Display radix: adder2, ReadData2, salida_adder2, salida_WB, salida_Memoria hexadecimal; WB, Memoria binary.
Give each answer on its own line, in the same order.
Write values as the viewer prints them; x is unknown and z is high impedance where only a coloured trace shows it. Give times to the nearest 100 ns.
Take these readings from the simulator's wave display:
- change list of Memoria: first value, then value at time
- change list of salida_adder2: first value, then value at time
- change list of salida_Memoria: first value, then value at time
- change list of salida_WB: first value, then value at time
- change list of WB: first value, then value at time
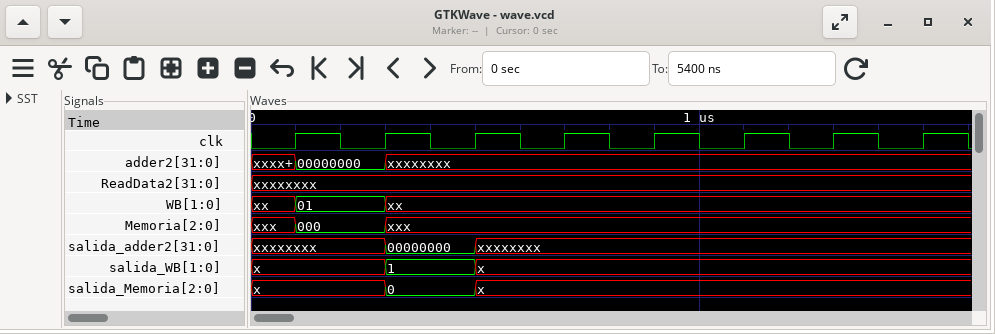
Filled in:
xxx, 000 at 100 ns, xxx at 300 ns
xxxxxxxx, 00000000 at 300 ns, xxxxxxxx at 500 ns
x, 0 at 300 ns, x at 500 ns
x, 1 at 300 ns, x at 500 ns
xx, 01 at 100 ns, xx at 300 ns
